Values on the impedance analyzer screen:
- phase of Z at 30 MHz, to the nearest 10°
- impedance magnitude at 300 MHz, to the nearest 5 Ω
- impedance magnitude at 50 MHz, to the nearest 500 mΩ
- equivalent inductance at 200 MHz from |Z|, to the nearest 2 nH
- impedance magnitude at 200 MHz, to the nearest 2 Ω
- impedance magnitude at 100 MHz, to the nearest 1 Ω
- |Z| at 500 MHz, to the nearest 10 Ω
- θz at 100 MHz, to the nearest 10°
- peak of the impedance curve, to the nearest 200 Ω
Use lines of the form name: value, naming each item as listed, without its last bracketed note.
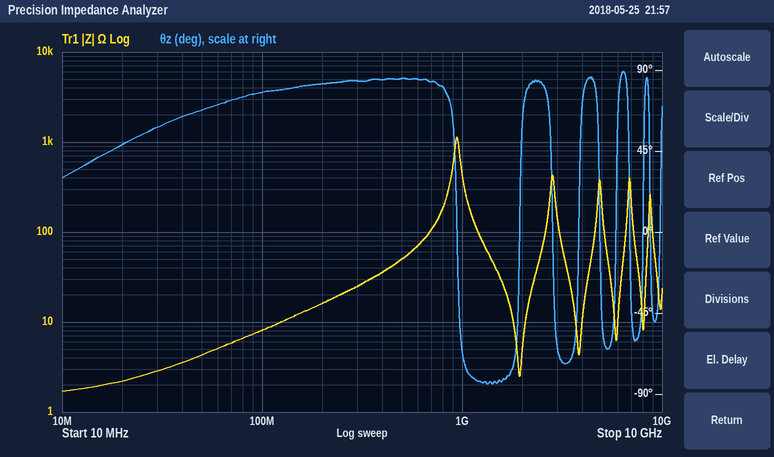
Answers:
phase of Z at 30 MHz, to the nearest 10°: 60°
impedance magnitude at 300 MHz, to the nearest 5 Ω: 25 Ω
impedance magnitude at 50 MHz, to the nearest 500 mΩ: 4.5 Ω
equivalent inductance at 200 MHz from |Z|, to the nearest 2 nH: 12 nH
impedance magnitude at 200 MHz, to the nearest 2 Ω: 16 Ω
impedance magnitude at 100 MHz, to the nearest 1 Ω: 8 Ω
|Z| at 500 MHz, to the nearest 10 Ω: 50 Ω
θz at 100 MHz, to the nearest 10°: 80°
peak of the impedance curve, to the nearest 200 Ω: 1.2 kΩ
